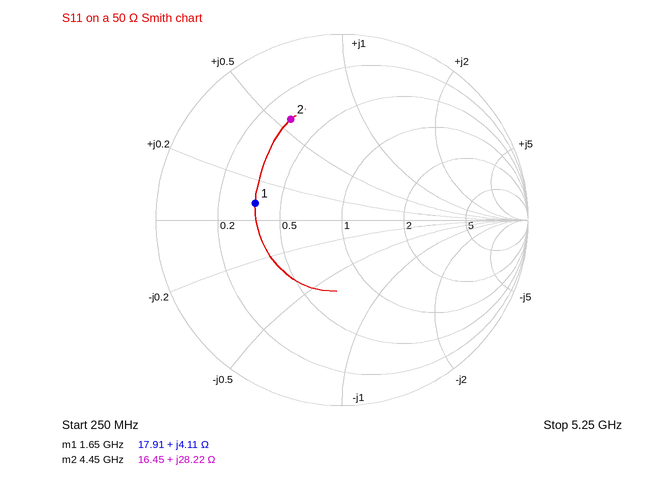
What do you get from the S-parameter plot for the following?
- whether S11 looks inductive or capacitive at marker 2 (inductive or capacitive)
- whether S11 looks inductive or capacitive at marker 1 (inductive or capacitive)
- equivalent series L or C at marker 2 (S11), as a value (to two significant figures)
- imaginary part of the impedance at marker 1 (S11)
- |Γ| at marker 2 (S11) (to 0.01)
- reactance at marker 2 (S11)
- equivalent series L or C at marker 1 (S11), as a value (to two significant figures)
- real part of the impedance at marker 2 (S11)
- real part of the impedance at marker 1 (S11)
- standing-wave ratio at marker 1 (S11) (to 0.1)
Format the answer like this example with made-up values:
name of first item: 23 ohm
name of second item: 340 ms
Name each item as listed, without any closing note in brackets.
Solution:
whether S11 looks inductive or capacitive at marker 2: inductive
whether S11 looks inductive or capacitive at marker 1: inductive
equivalent series L or C at marker 2 (S11), as a value: 1.0 nH
imaginary part of the impedance at marker 1: +4.11 Ω
|Γ| at marker 2 (S11): 0.61
reactance at marker 2: +28.22 Ω
equivalent series L or C at marker 1 (S11), as a value: 400 pH
real part of the impedance at marker 2: 16.45 Ω
real part of the impedance at marker 1: 17.91 Ω
standing-wave ratio at marker 1 (S11): 2.8
